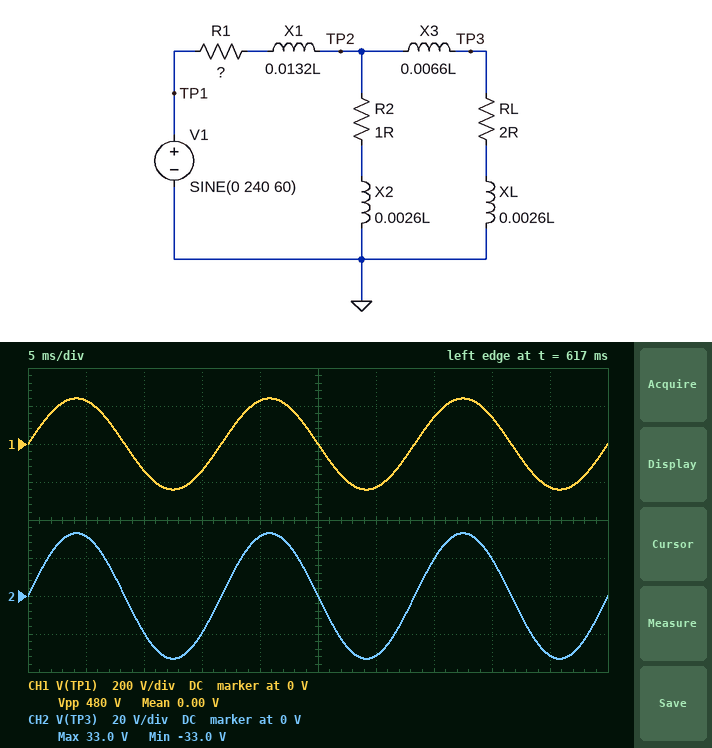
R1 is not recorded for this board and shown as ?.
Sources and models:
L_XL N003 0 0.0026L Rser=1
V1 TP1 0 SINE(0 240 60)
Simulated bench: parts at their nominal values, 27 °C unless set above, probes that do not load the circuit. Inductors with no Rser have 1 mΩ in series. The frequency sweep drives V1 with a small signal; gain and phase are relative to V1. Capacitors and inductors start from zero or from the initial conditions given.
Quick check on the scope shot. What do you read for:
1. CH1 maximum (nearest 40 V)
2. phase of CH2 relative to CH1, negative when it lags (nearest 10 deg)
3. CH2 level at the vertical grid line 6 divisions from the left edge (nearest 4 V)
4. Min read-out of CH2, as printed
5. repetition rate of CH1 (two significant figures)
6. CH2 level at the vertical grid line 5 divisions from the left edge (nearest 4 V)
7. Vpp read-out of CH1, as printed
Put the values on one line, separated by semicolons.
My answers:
240 V; 0 deg; -32 V; -33.0 V; 60 Hz; 0 V; 480 V
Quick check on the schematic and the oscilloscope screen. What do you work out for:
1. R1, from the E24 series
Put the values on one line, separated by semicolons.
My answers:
4.7 Ω
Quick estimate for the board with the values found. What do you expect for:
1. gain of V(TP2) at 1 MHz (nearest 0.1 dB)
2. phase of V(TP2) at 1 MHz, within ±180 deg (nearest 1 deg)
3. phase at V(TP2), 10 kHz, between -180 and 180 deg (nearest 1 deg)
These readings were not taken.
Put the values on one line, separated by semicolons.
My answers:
-17.5 dB; 0 deg; 0 deg
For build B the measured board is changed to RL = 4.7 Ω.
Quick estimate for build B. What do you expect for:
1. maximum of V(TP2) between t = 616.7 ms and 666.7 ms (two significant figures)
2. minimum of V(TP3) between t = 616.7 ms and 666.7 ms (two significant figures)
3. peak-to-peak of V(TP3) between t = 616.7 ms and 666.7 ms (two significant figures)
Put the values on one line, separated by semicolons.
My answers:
37 V; -37 V; 74 V
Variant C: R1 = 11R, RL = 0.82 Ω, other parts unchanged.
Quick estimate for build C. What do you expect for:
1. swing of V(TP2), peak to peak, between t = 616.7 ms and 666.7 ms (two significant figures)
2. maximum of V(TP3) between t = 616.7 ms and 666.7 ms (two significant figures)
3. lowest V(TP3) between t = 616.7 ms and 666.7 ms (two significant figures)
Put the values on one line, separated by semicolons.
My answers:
27 V; 13 V; -13 V
